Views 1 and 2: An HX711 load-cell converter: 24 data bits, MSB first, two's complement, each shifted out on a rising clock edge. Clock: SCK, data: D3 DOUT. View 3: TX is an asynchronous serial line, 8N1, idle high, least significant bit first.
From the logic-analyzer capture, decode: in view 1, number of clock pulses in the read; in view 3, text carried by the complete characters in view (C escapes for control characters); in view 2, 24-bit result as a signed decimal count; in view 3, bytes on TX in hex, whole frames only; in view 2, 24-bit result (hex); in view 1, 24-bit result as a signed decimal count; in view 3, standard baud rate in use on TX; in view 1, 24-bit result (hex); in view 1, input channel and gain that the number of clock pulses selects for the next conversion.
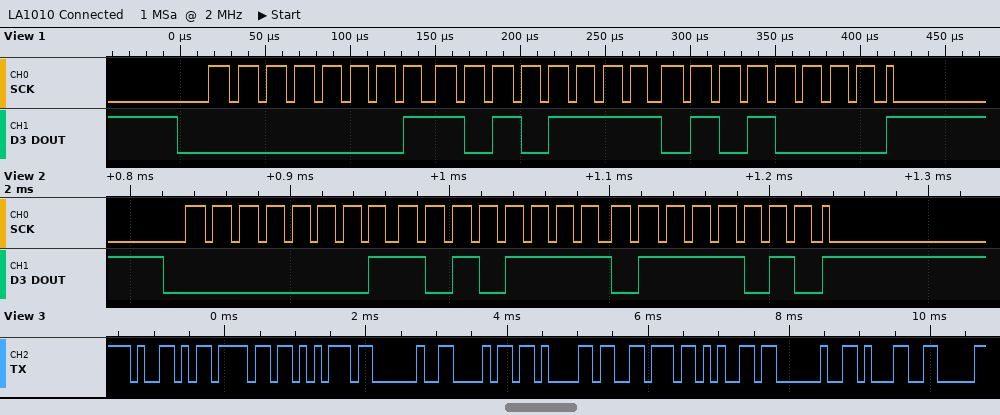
25
"You have 1"
110458
59 6F 75 20 68 61 76 65 20 31
0x01AF7A
110416
9600 baud
0x01AF50
channel A, gain 128
